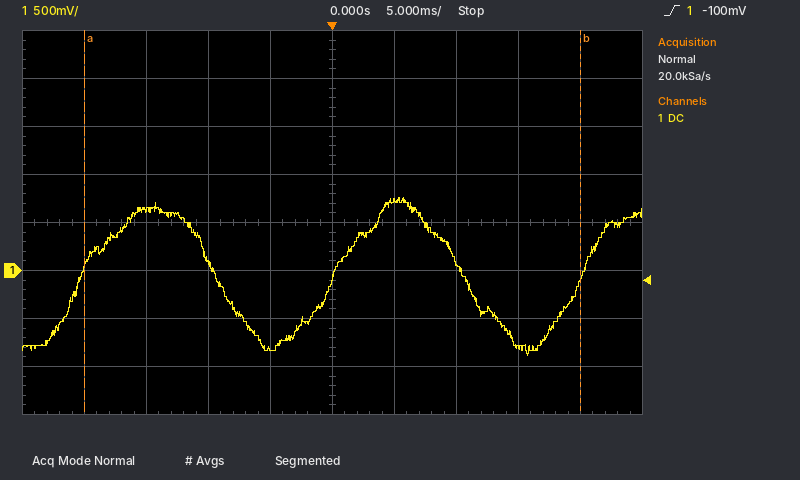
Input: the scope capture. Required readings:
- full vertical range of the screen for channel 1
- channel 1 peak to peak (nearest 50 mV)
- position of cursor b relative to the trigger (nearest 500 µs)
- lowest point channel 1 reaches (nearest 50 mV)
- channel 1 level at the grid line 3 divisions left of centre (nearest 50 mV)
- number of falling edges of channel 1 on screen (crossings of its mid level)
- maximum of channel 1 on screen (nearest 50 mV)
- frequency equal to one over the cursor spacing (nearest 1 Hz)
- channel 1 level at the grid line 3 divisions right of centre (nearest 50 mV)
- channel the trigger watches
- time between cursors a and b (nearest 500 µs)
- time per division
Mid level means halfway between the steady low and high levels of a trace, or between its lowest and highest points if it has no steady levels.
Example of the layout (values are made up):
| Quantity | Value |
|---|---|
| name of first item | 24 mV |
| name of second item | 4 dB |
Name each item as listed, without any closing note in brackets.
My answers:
| Quantity | Value |
|---|---|
| full vertical range of the screen for channel 1 | 4 V |
| channel 1 peak to peak | 1.65 V |
| position of cursor b relative to the trigger | +20.0 ms |
| lowest point channel 1 reaches | -900 mV |
| channel 1 level at the grid line 3 divisions left of centre | 650 mV |
| number of falling edges of channel 1 on screen | 2 |
| maximum of channel 1 on screen | 750 mV |
| frequency equal to one over the cursor spacing | 25 Hz |
| channel 1 level at the grid line 3 divisions right of centre | -800 mV |
| channel the trigger watches | channel 1 |
| time between cursors a and b | 40.0 ms |
| time per division | 5 ms |
